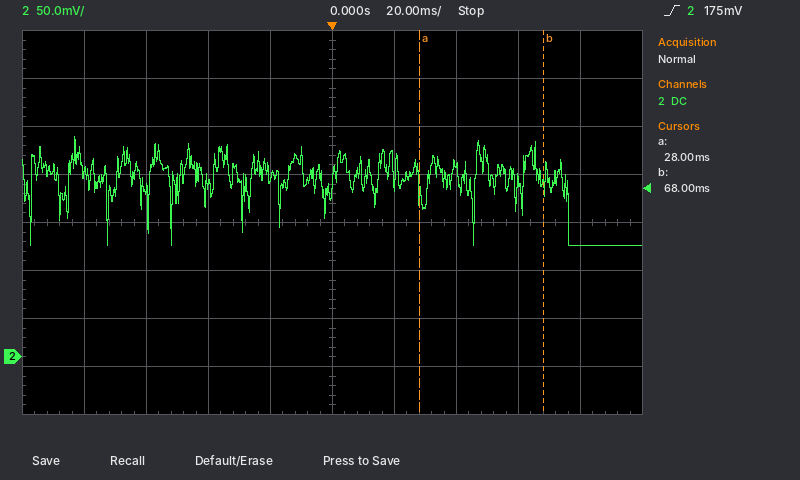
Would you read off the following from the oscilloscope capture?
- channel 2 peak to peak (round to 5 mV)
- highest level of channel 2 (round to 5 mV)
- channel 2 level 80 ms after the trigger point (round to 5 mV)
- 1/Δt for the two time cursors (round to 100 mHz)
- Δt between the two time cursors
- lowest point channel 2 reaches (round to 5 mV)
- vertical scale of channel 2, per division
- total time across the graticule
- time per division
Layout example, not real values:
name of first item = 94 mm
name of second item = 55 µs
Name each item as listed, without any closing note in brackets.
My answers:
channel 2 peak to peak = 115 mV
highest level of channel 2 = 230 mV
channel 2 level 80 ms after the trigger point = 115 mV
1/Δt for the two time cursors = 25.0 Hz
Δt between the two time cursors = 40 ms
lowest point channel 2 reaches = 115 mV
vertical scale of channel 2, per division = 50 mV
total time across the graticule = 200 ms
time per division = 20 ms
